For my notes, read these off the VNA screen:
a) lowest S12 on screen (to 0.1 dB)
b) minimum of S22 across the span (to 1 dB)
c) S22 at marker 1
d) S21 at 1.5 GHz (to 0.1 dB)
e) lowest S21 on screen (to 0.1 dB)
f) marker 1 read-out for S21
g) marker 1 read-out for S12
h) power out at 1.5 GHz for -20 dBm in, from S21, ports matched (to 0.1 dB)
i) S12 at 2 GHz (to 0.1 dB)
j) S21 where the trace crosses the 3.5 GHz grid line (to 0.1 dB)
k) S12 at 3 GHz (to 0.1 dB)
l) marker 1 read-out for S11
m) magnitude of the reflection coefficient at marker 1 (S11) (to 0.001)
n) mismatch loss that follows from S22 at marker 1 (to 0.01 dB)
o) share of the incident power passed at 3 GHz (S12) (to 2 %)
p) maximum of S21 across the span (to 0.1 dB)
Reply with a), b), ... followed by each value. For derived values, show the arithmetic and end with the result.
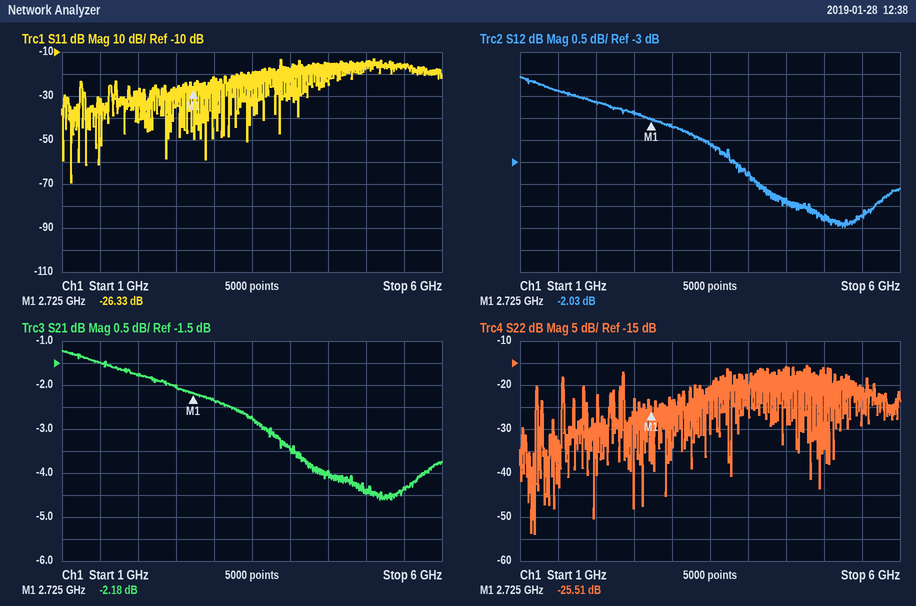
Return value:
a) -4.5 dB
b) -54 dB
c) -25.51 dB
d) -1.5 dB
e) -4.6 dB
f) -2.18 dB
g) -2.03 dB
h) -20 dBm + (-1.5 dB) = -21.5 dBm
i) -1.6 dB
j) -2.7 dB
k) -2.2 dB
l) -26.33 dB
m) 10^(-26.33/20) ≈ 0.048
n) −10 log10(1 − 10^(-25.51/10)) ≈ 0.01 dB
o) 10^(-2.2/10) ≈ 60 %
p) -1.2 dB
